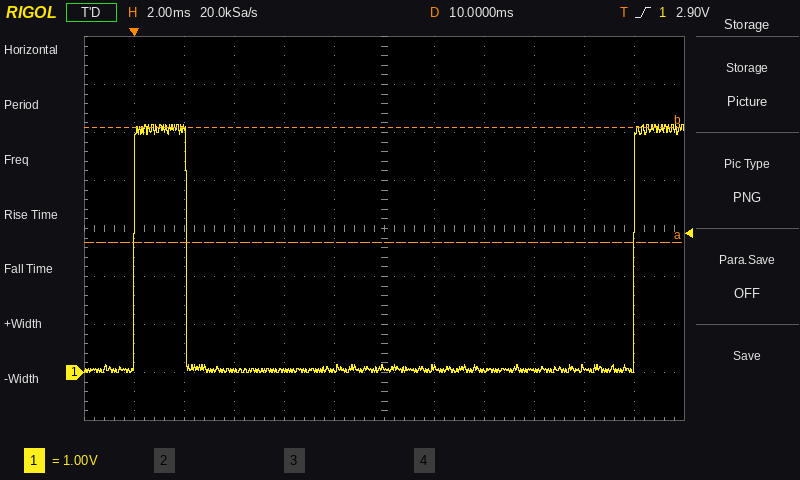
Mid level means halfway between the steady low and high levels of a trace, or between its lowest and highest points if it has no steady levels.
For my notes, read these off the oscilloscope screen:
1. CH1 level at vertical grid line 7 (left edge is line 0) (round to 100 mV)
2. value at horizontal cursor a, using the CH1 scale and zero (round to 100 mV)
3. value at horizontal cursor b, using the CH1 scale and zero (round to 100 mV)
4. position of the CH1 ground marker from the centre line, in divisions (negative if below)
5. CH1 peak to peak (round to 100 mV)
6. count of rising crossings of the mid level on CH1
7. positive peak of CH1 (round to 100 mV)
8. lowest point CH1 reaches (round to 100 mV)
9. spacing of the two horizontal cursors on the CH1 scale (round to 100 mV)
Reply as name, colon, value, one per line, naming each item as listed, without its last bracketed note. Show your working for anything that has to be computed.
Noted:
CH1 level at vertical grid line 7 (left edge is line 0): 100 mV
value at horizontal cursor a, using the CH1 scale and zero: 2.7 V
value at horizontal cursor b, using the CH1 scale and zero: 5.1 V
position of the CH1 ground marker from the centre line, in divisions: -3.0 div
CH1 peak to peak: 5.2 V − (0.0 V) = 5.2 V
count of rising crossings of the mid level on CH1: 2
positive peak of CH1: 5.2 V
lowest point CH1 reaches: 0.0 V
spacing of the two horizontal cursors on the CH1 scale: 2.4 V
